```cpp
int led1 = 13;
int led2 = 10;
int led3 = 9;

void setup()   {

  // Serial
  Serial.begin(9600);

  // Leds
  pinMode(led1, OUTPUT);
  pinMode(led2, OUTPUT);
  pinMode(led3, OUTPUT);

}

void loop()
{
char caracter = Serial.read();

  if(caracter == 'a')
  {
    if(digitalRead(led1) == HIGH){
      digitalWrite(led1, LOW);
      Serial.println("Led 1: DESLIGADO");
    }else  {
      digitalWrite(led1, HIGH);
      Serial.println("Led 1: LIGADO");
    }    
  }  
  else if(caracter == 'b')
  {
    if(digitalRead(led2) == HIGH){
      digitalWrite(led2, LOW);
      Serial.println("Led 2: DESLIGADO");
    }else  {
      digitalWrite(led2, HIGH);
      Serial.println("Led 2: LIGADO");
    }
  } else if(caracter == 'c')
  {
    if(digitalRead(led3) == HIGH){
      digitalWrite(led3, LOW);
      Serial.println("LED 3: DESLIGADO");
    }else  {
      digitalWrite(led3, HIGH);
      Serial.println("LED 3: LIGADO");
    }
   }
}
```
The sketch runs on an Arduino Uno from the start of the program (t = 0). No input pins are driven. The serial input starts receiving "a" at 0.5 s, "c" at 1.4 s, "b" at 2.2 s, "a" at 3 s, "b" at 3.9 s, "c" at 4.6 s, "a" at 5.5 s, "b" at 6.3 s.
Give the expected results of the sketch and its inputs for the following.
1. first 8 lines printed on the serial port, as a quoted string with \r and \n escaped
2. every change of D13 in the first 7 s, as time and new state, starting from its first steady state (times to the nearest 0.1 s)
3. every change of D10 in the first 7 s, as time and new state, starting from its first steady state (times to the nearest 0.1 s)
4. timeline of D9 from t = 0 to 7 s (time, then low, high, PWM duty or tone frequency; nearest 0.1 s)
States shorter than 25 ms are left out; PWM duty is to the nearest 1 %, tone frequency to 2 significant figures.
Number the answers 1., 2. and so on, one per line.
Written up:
1. "Led 1: LIGADO\r\nLED 3: LIGADO\r\nLed 2: LIGADO\r\nLed 1: DESLIGADO\r\nLed 2: DESLIGADO\r\nLED 3: DESLIGADO\r\nLed 1: LIGADO\r\nLed 2: LIGADO\r\n"
2. 0 s low; 0.5 s high; 3 s low; 5.5 s high
3. 0 s low; 2.2 s high; 3.9 s low; 6.3 s high
4. 0 s low; 1.4 s high; 4.6 s low
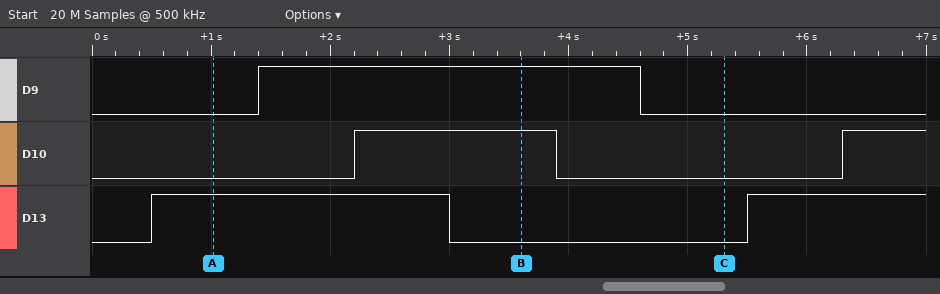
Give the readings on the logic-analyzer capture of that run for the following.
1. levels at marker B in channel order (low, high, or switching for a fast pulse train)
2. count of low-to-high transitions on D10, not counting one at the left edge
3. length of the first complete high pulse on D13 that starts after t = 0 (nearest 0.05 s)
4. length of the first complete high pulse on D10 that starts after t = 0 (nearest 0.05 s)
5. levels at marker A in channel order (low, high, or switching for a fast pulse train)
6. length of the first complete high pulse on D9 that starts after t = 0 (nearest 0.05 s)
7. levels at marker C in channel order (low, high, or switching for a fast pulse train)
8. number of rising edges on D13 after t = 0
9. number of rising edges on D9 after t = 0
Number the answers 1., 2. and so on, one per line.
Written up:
1. D9 high, D10 high, D13 low
2. 2
3. 2.50 s
4. 1.70 s
5. D9 low, D10 low, D13 high
6. 3.20 s
7. D9 low, D10 low, D13 low
8. 2
9. 1
